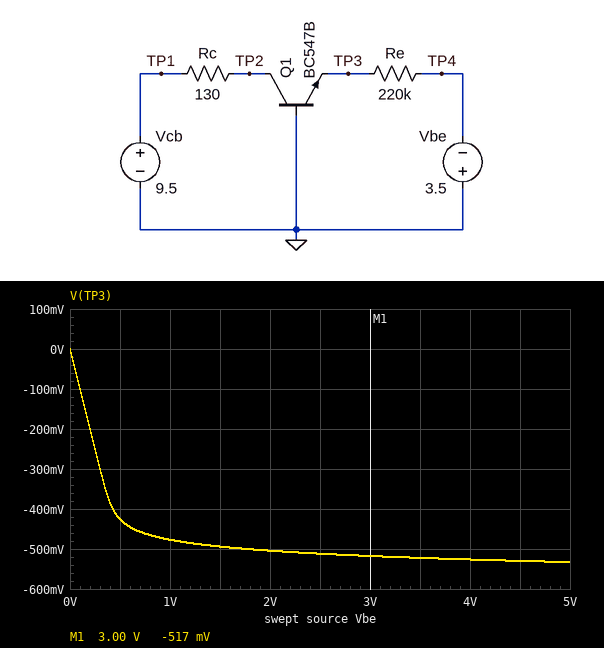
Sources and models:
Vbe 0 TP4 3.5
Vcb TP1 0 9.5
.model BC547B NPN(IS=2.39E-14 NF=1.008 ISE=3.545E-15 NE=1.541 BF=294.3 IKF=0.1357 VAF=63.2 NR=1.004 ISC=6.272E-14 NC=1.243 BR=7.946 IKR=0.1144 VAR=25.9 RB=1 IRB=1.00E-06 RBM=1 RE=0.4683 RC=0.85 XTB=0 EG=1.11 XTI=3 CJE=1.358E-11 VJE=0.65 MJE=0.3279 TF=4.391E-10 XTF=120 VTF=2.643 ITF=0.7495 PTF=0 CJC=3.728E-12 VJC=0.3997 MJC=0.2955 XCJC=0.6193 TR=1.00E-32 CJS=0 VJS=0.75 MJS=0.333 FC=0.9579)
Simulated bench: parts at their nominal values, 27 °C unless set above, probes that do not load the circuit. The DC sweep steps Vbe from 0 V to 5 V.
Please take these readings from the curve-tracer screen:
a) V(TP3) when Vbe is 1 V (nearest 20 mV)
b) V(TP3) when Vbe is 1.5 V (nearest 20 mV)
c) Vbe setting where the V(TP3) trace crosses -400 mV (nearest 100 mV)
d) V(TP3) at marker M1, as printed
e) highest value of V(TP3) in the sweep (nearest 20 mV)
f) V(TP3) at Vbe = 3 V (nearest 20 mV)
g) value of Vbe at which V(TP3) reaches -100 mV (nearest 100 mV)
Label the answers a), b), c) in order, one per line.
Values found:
a) -480 mV
b) -500 mV
c) 400 mV
d) -517 mV
e) 0 V
f) -520 mV
g) 100 mV
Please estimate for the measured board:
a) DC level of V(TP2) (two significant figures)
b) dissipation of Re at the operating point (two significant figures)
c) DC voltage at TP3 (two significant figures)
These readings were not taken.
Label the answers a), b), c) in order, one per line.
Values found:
a) 9.5 V
b) 40 µW
c) -520 mV
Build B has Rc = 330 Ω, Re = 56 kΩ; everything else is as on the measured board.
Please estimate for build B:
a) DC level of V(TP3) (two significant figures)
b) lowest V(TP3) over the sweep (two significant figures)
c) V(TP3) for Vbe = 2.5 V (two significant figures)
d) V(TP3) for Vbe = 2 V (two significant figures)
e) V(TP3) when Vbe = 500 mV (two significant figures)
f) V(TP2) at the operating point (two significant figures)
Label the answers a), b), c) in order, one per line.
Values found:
a) -560 mV
b) -570 mV
c) -550 mV
d) -540 mV
e) -450 mV
f) 9.5 V
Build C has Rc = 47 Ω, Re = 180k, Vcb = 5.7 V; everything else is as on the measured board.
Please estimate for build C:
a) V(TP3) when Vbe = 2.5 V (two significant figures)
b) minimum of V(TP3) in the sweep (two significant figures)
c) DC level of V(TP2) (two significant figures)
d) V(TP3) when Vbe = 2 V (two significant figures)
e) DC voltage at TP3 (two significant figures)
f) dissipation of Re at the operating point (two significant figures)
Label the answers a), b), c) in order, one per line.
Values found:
a) -520 mV
b) -540 mV
c) 5.7 V
d) -510 mV
e) -530 mV
f) 49 µW
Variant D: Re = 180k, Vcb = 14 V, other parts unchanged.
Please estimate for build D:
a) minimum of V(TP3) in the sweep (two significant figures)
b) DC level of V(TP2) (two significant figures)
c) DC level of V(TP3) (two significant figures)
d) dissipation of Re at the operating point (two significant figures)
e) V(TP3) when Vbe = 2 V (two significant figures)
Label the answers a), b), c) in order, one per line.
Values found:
a) -540 mV
b) 14 V
c) -530 mV
d) 49 µW
e) -510 mV
